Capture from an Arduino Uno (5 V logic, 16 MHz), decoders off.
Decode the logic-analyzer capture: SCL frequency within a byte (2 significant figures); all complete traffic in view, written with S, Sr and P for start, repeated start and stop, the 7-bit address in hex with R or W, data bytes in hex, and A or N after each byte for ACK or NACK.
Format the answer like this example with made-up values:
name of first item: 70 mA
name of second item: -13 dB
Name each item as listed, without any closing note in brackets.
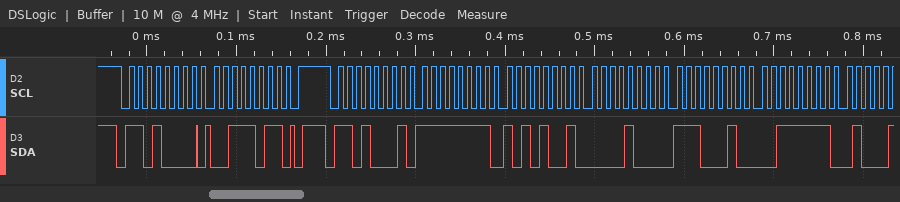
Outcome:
SCL frequency within a byte: 100 kHz
all complete traffic in view, written with S, Sr and P for start, repeated start and stop, the 7-bit address in hex with R or W, data bytes in hex, and A or N after each byte for ACK or NACK: S 68W A 3B A P S 68R A FF A A9 A 08 A E2 A 3F A
